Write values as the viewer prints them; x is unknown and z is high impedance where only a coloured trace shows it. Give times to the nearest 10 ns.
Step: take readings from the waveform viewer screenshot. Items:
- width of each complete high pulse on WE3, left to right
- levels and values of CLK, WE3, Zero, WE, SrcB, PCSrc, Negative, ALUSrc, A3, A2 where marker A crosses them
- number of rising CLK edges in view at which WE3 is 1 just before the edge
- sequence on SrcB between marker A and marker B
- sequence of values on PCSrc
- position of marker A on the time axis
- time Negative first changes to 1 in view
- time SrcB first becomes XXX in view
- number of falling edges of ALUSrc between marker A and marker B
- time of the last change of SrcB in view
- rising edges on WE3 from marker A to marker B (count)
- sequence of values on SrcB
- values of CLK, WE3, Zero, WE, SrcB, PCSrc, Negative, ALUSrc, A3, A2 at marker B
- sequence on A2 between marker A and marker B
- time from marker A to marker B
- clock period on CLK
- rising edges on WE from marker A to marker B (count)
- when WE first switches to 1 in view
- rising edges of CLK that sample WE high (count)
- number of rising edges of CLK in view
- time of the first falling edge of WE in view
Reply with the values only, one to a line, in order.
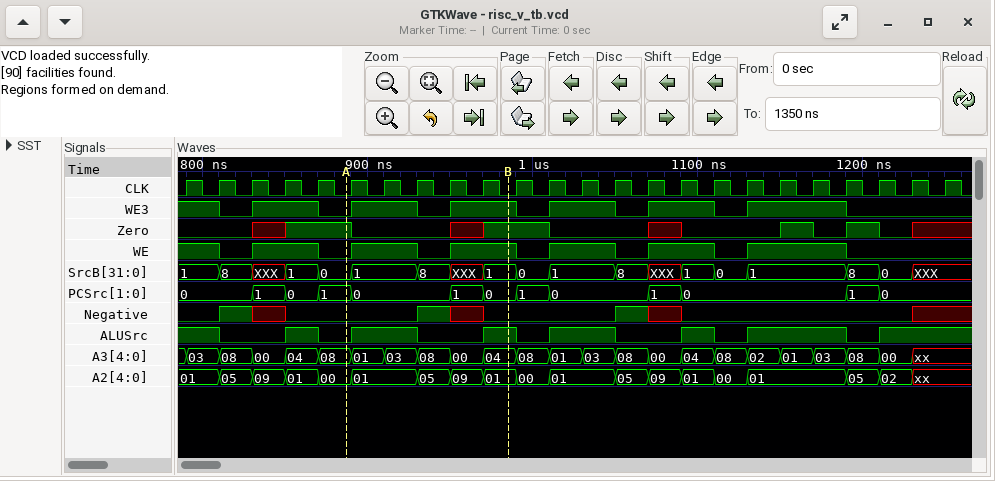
40 ns, 40 ns, 40 ns, 40 ns, 40 ns, 60 ns
CLK=0, WE3=0, Zero=1, WE=0, SrcB=0, PCSrc=1, Negative=0, ALUSrc=0, A3=08, A2=00
15
0, 1, 8, XXX, 1
0, 1, 0, 1, 0, 1, 0, 1, 0, 1, 0, 1, 0
890 ns
810 ns
830 ns
1
1230 ns
2
1, 8, XXX, 1, 0, 1, 8, XXX, 1, 0, 1, 8, XXX, 1, 0, 1, 8, 0, XXX
CLK=0, WE3=1, Zero=1, WE=1, SrcB=1, PCSrc=0, Negative=0, ALUSrc=1, A3=04, A2=01
00, 01, 05, 09, 01
100 ns
20 ns
2
830 ns
15
24
810 ns
